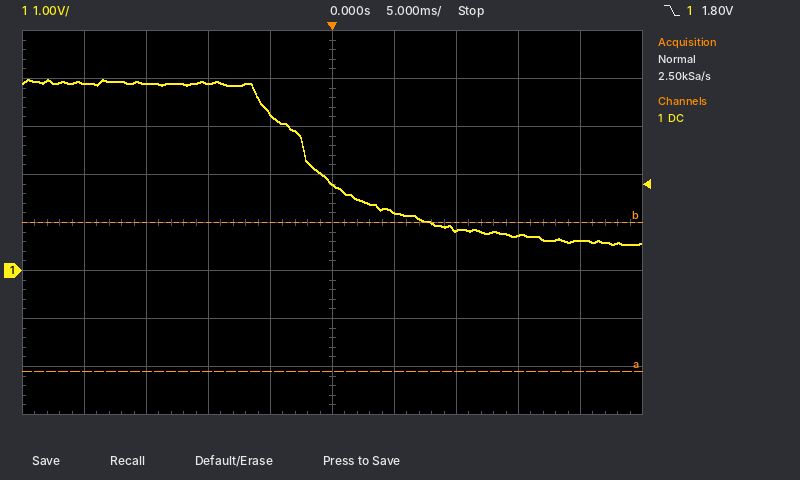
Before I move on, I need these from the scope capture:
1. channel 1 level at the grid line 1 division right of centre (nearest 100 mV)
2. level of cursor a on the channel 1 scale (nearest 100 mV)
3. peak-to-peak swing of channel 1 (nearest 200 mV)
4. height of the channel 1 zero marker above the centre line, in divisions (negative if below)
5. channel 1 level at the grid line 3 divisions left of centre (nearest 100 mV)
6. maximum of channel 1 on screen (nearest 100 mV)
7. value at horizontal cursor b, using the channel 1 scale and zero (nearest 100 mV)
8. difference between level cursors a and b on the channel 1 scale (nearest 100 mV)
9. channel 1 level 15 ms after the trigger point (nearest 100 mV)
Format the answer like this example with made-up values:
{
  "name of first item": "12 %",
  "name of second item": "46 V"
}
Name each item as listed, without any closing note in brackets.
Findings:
{
  "channel 1 level at the grid line 1 division right of centre": "1.2 V",
  "level of cursor a on the channel 1 scale": "-2.1 V",
  "peak-to-peak swing of channel 1": "3.4 V",
  "height of the channel 1 zero marker above the centre line, in divisions": "-1.0 div",
  "channel 1 level at the grid line 3 divisions left of centre": "3.9 V",
  "maximum of channel 1 on screen": "4.0 V",
  "value at horizontal cursor b, using the channel 1 scale and zero": "1.0 V",
  "difference between level cursors a and b on the channel 1 scale": "3.1 V",
  "channel 1 level 15 ms after the trigger point": "700 mV"
}
